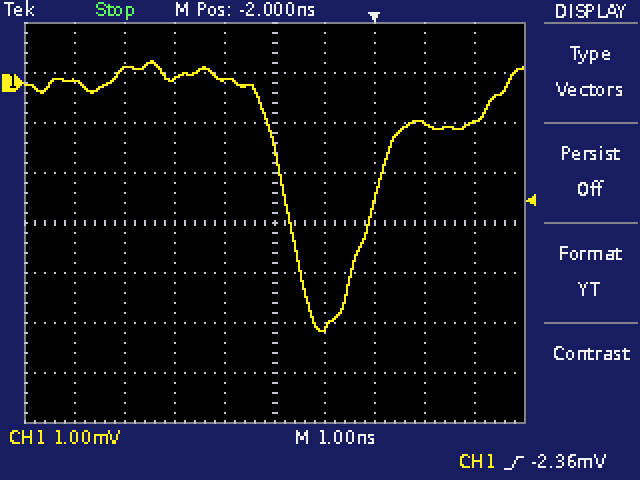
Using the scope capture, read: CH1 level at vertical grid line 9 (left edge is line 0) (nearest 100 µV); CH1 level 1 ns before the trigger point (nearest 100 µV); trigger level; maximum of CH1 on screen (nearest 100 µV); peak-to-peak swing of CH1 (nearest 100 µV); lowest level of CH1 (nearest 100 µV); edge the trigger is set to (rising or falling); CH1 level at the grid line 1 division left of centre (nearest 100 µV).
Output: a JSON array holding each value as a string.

["-800 µV", "-4.9 mV", "-2.36 mV", "400 µV", "5.4 mV", "-5.0 mV", "rising", "100 µV"]
